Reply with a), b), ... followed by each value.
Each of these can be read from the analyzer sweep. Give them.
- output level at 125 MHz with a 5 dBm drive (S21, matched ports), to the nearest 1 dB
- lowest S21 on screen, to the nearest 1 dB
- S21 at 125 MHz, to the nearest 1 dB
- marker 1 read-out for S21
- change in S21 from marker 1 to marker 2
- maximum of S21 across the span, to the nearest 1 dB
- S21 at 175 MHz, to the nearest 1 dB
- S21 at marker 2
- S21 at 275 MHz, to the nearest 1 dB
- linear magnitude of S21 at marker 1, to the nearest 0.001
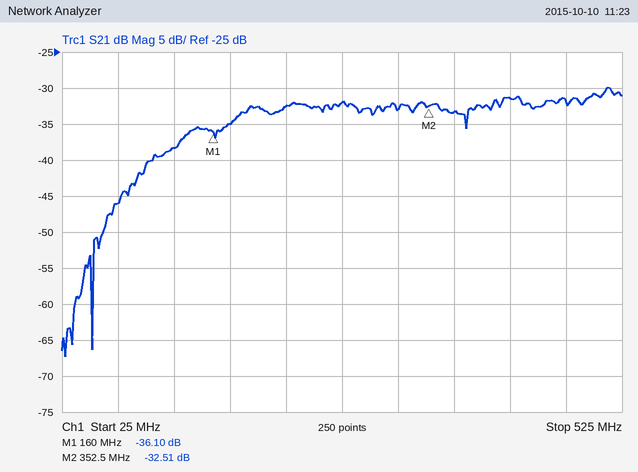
a) -33 dBm
b) -67 dB
c) -38 dB
d) -36.10 dB
e) 3.59 dB
f) -30 dB
g) -35 dB
h) -32.51 dB
i) -32 dB
j) 0.016
